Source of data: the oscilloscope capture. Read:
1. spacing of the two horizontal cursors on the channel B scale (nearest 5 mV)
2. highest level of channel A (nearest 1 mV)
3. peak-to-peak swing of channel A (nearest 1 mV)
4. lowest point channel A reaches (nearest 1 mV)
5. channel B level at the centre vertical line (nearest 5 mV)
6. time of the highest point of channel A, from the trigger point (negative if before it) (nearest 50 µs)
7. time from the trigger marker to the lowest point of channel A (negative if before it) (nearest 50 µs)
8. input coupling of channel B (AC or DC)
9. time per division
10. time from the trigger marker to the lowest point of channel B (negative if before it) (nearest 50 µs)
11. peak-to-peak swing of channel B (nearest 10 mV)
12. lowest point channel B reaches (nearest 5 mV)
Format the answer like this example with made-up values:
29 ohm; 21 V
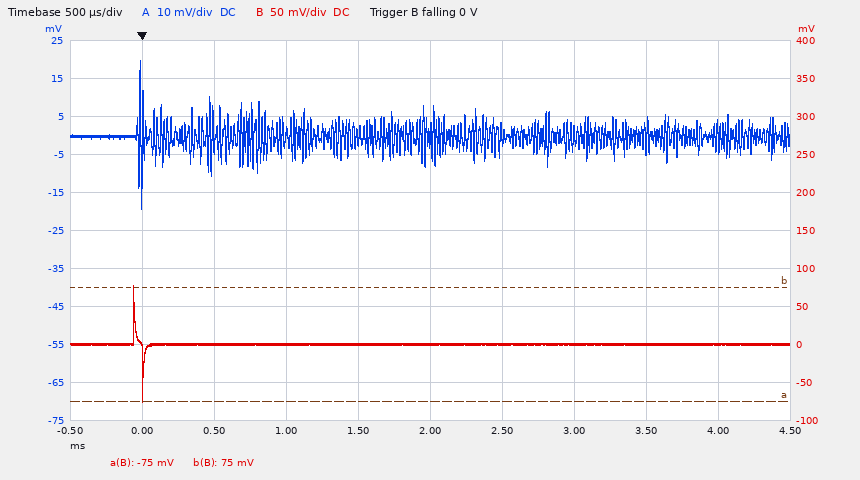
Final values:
150 mV; 20 mV; 39 mV; -19 mV; 0 mV; 0 µs; 0 µs; DC; 500 µs; 0 µs; 150 mV; -75 mV
